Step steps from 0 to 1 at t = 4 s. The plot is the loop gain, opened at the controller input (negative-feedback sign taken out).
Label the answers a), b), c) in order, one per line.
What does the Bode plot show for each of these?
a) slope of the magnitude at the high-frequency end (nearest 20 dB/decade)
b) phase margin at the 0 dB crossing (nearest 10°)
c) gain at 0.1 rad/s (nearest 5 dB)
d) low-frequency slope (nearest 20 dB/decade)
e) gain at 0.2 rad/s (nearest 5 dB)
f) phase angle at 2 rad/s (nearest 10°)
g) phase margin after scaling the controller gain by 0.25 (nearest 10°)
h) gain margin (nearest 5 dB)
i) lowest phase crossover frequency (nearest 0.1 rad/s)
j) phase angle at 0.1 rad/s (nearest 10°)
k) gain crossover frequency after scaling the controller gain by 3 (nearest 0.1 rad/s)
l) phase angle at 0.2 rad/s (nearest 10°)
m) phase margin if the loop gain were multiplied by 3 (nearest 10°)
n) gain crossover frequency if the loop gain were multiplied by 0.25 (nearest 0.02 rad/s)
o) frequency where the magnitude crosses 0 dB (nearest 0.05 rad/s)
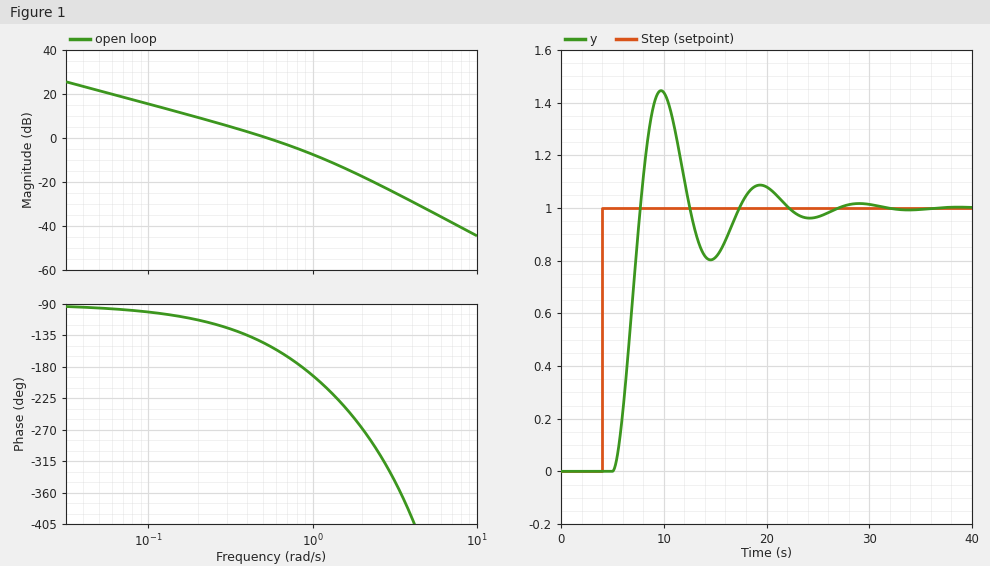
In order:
a) -40 dB/decade
b) 30°
c) 15 dB
d) -20 dB/decade
e) 10 dB
f) -270°
g) 70°
h) 5 dB
i) 0.9 rad/s
j) -100°
k) 1.2 rad/s
l) -110°
m) -30°
n) 0.14 rad/s
o) 0.55 rad/s
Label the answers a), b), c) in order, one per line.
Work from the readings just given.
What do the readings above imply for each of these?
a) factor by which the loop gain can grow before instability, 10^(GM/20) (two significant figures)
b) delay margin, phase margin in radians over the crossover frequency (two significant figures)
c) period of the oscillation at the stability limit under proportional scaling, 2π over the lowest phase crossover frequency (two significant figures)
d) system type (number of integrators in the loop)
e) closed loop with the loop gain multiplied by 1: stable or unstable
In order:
a) 1.8
b) 0.95 s
c) 7.0 s
d) 1
e) stable
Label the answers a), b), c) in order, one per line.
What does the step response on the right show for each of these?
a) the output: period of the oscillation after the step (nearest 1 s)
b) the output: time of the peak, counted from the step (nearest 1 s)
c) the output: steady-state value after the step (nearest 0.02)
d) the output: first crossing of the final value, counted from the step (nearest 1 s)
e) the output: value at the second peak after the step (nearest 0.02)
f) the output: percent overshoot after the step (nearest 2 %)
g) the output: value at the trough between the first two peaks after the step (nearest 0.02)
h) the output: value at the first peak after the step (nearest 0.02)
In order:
a) 10 s
b) 6 s
c) 1.00
d) 4 s
e) 1.08
f) 44 %
g) 0.80
h) 1.44
